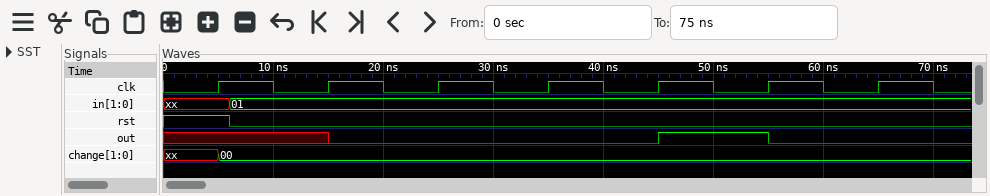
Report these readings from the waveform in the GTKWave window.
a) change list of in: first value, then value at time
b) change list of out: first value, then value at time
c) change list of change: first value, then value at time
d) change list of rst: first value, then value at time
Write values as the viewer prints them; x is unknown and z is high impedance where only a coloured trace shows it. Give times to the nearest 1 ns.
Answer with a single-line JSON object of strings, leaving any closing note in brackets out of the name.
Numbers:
{"change list of in: first value, then value at time": "xx, 01 at 6 ns", "change list of out: first value, then value at time": "x, 0 at 15 ns, 1 at 45 ns, 0 at 55 ns", "change list of change: first value, then value at time": "xx, 00 at 5 ns", "change list of rst: first value, then value at time": "1, 0 at 6 ns"}
